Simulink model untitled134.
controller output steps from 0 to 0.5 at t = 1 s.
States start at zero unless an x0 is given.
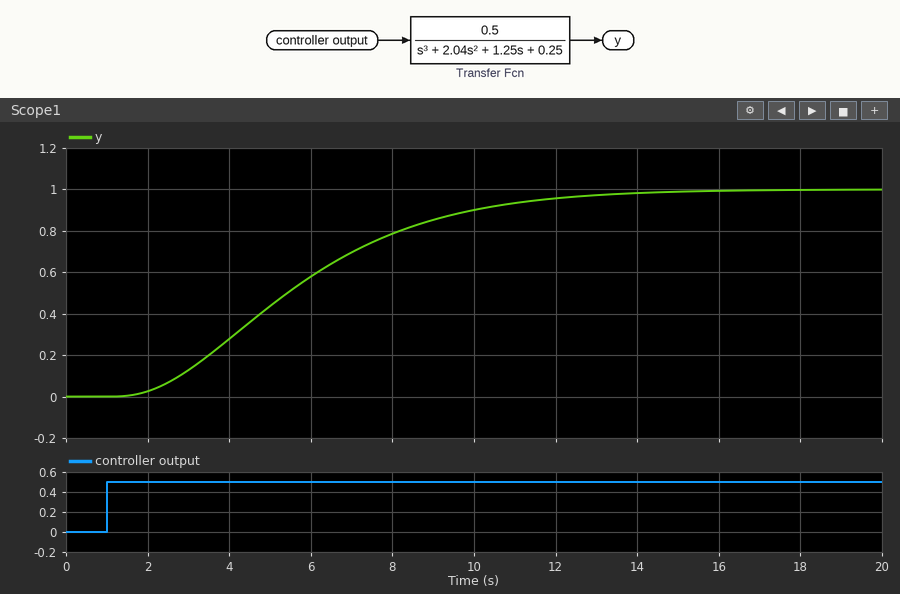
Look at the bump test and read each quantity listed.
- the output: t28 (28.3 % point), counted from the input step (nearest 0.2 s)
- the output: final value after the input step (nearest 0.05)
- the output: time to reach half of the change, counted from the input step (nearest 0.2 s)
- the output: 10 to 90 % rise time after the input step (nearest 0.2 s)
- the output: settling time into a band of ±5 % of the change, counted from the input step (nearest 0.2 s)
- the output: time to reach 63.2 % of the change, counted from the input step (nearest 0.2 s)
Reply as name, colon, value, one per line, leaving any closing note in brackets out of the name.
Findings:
the output: t28 (28.3 % point), counted from the input step: 3.0 s
the output: final value after the input step: 1.00
the output: time to reach half of the change, counted from the input step: 4.4 s
the output: 10 to 90 % rise time after the input step: 7.2 s
the output: settling time into a band of ±5 % of the change, counted from the input step: 10.6 s
the output: time to reach 63.2 % of the change, counted from the input step: 5.4 s
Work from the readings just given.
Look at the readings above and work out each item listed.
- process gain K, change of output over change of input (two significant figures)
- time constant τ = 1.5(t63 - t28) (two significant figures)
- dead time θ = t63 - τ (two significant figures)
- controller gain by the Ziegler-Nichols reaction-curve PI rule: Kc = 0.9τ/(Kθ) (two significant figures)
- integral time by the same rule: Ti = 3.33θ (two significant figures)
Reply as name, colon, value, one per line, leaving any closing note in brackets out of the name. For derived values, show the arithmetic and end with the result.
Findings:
process gain K, change of output over change of input: (1 - 0) / 0.5 = 2.0
time constant τ = 1.5(t63 - t28): 1.5 × (5.4 - 3) = 3.6 s
dead time θ = t63 - τ: 5.4 - 3.6 = 1.8 s
controller gain by the Ziegler-Nichols reaction-curve PI rule: Kc = 0.9τ/(Kθ): 0.9 × 3.6 / (2 × 1.8) = 0.90
integral time by the same rule: Ti = 3.33θ: 3.33 × 1.8 = 6.0 s
